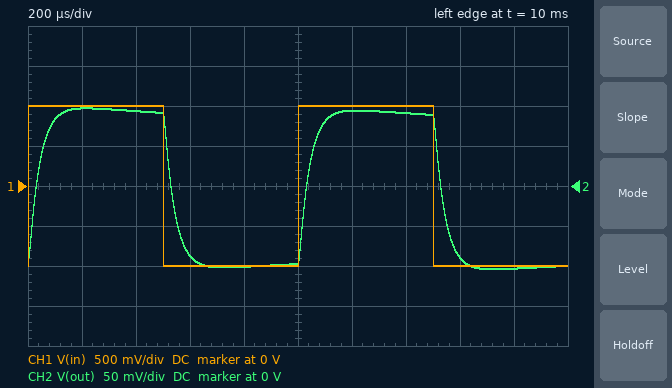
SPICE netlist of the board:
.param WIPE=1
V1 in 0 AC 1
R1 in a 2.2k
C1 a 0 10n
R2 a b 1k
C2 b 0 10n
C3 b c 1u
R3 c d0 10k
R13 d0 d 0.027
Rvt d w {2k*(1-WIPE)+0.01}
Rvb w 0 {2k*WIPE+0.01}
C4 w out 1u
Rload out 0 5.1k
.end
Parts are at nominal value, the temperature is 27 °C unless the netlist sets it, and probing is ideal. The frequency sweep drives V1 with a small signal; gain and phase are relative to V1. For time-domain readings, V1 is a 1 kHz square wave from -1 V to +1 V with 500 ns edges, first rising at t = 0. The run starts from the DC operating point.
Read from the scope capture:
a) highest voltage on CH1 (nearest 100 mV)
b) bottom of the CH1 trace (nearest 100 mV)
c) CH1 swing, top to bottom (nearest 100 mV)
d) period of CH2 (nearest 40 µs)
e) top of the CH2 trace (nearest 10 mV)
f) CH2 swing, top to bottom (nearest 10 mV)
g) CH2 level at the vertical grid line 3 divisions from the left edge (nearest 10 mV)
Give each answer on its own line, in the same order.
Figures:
1.0 V
-1.0 V
2.0 V
1.00 ms
100 mV
200 mV
-90 mV
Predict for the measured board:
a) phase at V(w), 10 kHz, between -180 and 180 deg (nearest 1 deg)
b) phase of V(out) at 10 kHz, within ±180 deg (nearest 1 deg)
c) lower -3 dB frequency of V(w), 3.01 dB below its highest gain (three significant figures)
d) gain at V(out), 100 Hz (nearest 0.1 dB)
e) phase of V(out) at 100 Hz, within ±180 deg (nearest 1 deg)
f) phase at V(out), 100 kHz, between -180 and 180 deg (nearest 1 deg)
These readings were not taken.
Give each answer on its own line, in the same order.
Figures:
-83 deg
-83 deg
7.46 Hz
-20.5 dB
18 deg
-158 deg
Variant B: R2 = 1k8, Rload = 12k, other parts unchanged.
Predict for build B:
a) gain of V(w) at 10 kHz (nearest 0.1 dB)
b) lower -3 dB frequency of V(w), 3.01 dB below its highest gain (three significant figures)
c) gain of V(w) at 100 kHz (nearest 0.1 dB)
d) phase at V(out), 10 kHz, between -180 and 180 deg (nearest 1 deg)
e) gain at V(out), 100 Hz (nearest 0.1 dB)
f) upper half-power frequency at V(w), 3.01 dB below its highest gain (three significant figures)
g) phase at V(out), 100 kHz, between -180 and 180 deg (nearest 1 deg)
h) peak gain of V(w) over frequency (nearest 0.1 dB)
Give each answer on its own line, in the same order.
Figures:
-29.0 dB
8.46 Hz
-60.8 dB
-93 deg
-19.4 dB
3.74 kHz
-165 deg
-19.3 dB
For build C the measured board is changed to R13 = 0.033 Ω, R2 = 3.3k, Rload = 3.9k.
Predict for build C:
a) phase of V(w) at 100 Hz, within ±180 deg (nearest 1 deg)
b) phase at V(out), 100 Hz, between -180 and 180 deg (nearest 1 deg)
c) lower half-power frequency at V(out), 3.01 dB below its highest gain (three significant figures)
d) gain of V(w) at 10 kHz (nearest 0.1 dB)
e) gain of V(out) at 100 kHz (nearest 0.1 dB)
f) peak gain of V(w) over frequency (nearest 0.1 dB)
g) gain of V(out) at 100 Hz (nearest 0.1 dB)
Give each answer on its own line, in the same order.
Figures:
-3 deg
19 deg
30.6 Hz
-33.3 dB
-67.9 dB
-20.6 dB
-22.5 dB
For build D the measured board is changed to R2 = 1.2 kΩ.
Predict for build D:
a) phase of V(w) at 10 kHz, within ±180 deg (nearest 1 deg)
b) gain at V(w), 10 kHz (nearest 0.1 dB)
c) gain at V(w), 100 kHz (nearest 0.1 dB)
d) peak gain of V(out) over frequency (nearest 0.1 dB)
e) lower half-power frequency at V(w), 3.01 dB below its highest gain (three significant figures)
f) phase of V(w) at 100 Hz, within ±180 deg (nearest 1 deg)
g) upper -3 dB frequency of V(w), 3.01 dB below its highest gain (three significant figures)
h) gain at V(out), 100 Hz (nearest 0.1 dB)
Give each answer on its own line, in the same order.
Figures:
-86 deg
-29.3 dB
-58.8 dB
-20.3 dB
7.38 Hz
0 deg
3.39 kHz
-20.6 dB
